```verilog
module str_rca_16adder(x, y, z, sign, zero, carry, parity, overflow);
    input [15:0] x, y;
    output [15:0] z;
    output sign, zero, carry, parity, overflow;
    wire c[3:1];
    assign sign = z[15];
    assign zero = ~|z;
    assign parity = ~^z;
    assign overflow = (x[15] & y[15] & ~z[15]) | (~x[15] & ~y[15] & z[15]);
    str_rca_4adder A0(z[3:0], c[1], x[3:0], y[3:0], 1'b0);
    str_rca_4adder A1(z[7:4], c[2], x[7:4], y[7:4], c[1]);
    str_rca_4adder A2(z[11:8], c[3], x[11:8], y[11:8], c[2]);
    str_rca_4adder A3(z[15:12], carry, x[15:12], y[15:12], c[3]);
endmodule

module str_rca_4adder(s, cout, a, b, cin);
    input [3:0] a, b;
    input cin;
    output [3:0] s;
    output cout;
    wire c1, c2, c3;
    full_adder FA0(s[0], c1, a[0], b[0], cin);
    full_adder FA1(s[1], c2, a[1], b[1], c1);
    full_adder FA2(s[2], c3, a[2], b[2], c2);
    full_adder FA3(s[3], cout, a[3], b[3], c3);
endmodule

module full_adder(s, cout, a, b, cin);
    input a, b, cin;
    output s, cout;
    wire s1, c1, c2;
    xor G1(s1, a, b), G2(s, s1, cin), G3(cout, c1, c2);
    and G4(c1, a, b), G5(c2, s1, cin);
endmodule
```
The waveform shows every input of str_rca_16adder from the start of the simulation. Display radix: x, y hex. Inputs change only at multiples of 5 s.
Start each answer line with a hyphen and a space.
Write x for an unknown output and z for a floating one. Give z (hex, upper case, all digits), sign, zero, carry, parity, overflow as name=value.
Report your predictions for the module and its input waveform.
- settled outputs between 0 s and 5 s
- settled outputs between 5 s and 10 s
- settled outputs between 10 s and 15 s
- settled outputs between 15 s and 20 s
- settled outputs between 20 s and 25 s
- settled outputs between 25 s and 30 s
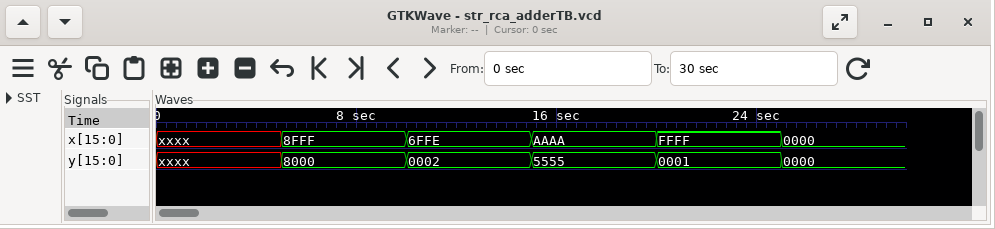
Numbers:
- z=x, sign=x, zero=x, carry=x, parity=x, overflow=x
- z=0FFF, sign=0, zero=0, carry=1, parity=1, overflow=1
- z=7000, sign=0, zero=0, carry=0, parity=0, overflow=0
- z=FFFF, sign=1, zero=0, carry=0, parity=1, overflow=0
- z=0000, sign=0, zero=1, carry=1, parity=1, overflow=0
- z=0000, sign=0, zero=1, carry=0, parity=1, overflow=0
